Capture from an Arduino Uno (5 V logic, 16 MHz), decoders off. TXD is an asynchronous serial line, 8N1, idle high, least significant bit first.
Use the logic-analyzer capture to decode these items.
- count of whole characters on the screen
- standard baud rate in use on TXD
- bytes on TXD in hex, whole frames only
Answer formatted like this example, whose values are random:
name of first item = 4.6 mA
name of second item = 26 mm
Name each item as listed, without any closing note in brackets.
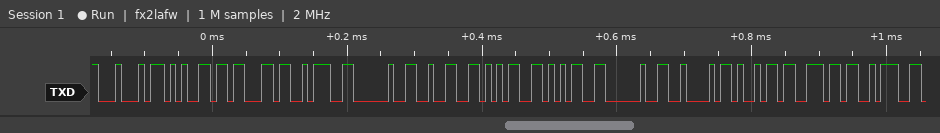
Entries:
count of whole characters on the screen = 13
standard baud rate in use on TXD = 115200 baud
bytes on TXD in hex, whole frames only = 0x44 0x65 0x63 0x3A 0x20 0x32 0x35 0x35 0x20 0x42 0x69 0x6E 0x3A
